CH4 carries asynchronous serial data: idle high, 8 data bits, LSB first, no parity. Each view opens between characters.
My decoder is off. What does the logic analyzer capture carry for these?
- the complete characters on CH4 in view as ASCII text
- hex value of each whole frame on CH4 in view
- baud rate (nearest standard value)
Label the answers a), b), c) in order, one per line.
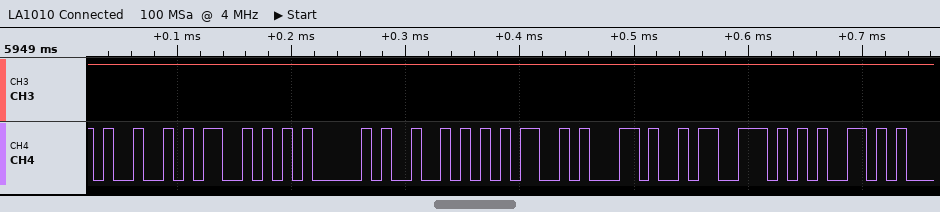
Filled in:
a) "ISARM,se"
b) 49, 53, 41, 52, 4D, 2C, 73, 65
c) 115200 baud
